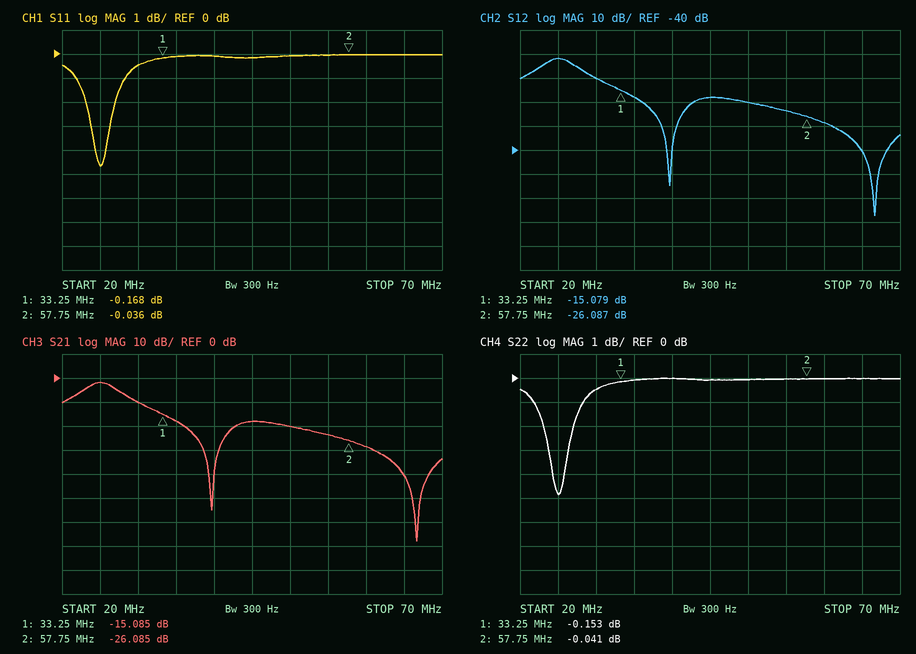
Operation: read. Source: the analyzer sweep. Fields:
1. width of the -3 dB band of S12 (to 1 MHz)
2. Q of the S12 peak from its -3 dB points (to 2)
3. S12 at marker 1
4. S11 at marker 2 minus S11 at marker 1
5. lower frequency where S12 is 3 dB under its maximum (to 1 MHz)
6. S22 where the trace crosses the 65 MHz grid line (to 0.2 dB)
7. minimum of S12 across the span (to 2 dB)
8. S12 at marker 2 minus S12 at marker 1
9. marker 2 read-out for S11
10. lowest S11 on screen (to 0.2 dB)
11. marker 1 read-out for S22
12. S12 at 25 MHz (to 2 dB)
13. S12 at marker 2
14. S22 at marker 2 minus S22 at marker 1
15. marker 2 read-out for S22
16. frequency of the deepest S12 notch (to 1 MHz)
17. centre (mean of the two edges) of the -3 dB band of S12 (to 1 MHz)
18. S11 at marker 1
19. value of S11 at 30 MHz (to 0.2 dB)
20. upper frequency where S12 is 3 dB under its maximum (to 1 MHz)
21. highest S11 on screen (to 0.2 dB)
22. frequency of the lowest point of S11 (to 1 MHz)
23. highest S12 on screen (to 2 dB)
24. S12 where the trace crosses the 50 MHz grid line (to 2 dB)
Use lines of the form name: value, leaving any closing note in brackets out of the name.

width of the -3 dB band of S12: 4 MHz
Q of the S12 peak from its -3 dB points: 6
S12 at marker 1: -15.079 dB
S11 at marker 2 minus S11 at marker 1: 0.132 dB
lower frequency where S12 is 3 dB under its maximum: 23 MHz
S22 where the trace crosses the 65 MHz grid line: 0.0 dB
minimum of S12 across the span: -68 dB
S12 at marker 2 minus S12 at marker 1: -11.008 dB
marker 2 read-out for S11: -0.036 dB
lowest S11 on screen: -4.6 dB
marker 1 read-out for S22: -0.153 dB
S12 at 25 MHz: -2 dB
S12 at marker 2: -26.087 dB
S22 at marker 2 minus S22 at marker 1: 0.112 dB
marker 2 read-out for S22: -0.041 dB
frequency of the deepest S12 notch: 67 MHz
centre (mean of the two edges) of the -3 dB band of S12: 25 MHz
S11 at marker 1: -0.168 dB
value of S11 at 30 MHz: -0.4 dB
upper frequency where S12 is 3 dB under its maximum: 27 MHz
highest S11 on screen: 0.0 dB
frequency of the lowest point of S11: 25 MHz
highest S12 on screen: -2 dB
S12 where the trace crosses the 50 MHz grid line: -20 dB
